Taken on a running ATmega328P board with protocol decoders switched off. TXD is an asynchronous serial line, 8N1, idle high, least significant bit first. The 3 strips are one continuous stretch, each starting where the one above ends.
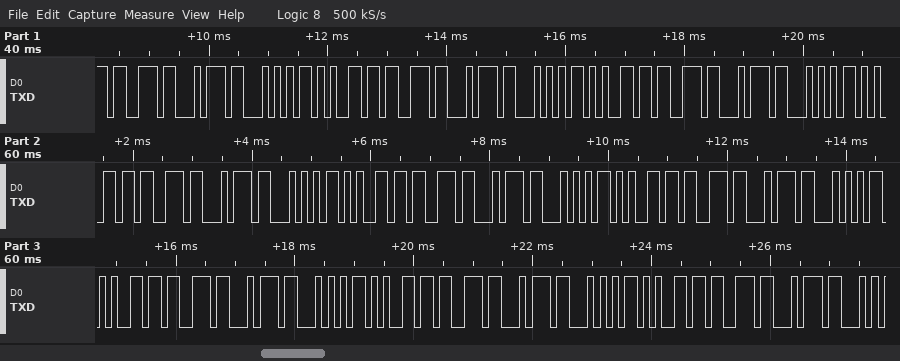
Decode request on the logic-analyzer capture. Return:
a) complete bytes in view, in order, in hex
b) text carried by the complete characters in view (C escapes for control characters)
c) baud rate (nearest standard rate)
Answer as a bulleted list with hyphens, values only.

- 73 74 54 65 73 74 54 65 73 74 54 65 73 74 54 65 73 74 54 65 73 74 54 65 73 74 54 65 73 74 54 65 73 74
- "stTestTestTestTestTestTestTestTest"
- 9600 baud
